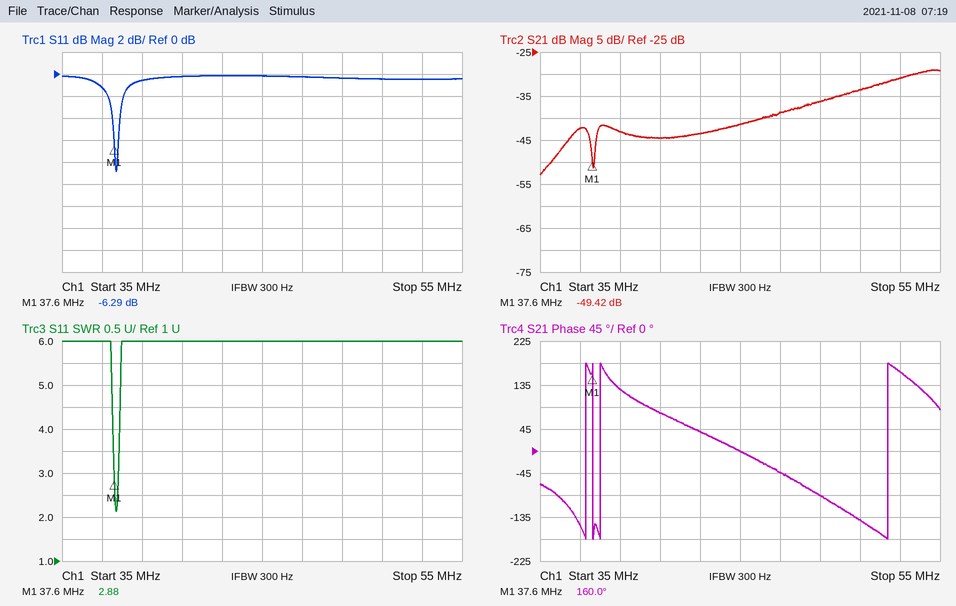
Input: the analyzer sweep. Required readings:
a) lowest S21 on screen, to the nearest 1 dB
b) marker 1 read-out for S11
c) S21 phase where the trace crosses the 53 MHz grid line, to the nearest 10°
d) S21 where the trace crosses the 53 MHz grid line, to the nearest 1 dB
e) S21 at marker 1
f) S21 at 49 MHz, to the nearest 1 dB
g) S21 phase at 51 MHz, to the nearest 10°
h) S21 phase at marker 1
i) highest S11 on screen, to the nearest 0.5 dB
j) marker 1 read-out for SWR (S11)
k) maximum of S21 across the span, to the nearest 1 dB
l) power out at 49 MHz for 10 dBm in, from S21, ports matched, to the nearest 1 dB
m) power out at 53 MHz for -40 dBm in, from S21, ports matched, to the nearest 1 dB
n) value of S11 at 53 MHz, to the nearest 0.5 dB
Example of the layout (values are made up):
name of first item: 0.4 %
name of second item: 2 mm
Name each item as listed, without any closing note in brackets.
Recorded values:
lowest S21 on screen, to the nearest 1 dB: -53 dB
marker 1 read-out for S11: -6.29 dB
S21 phase where the trace crosses the 53 MHz grid line, to the nearest 10°: 160°
S21 where the trace crosses the 53 MHz grid line, to the nearest 1 dB: -31 dB
S21 at marker 1: -49.42 dB
S21 at 49 MHz, to the nearest 1 dB: -36 dB
S21 phase at 51 MHz, to the nearest 10°: -140°
S21 phase at marker 1: 160.0°
highest S11 on screen, to the nearest 0.5 dB: 0.0 dB
marker 1 read-out for SWR: 2.88
maximum of S21 across the span, to the nearest 1 dB: -29 dB
power out at 49 MHz for 10 dBm in, from S21, ports matched, to the nearest 1 dB: -26 dBm
power out at 53 MHz for -40 dBm in, from S21, ports matched, to the nearest 1 dB: -71 dBm
value of S11 at 53 MHz, to the nearest 0.5 dB: -0.5 dB
